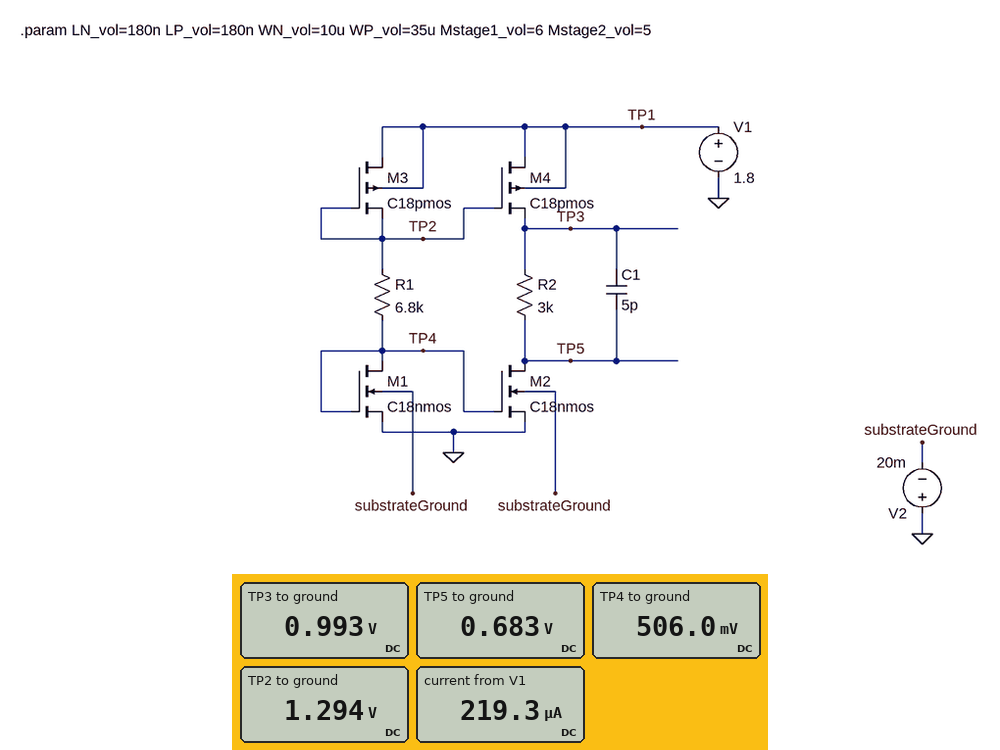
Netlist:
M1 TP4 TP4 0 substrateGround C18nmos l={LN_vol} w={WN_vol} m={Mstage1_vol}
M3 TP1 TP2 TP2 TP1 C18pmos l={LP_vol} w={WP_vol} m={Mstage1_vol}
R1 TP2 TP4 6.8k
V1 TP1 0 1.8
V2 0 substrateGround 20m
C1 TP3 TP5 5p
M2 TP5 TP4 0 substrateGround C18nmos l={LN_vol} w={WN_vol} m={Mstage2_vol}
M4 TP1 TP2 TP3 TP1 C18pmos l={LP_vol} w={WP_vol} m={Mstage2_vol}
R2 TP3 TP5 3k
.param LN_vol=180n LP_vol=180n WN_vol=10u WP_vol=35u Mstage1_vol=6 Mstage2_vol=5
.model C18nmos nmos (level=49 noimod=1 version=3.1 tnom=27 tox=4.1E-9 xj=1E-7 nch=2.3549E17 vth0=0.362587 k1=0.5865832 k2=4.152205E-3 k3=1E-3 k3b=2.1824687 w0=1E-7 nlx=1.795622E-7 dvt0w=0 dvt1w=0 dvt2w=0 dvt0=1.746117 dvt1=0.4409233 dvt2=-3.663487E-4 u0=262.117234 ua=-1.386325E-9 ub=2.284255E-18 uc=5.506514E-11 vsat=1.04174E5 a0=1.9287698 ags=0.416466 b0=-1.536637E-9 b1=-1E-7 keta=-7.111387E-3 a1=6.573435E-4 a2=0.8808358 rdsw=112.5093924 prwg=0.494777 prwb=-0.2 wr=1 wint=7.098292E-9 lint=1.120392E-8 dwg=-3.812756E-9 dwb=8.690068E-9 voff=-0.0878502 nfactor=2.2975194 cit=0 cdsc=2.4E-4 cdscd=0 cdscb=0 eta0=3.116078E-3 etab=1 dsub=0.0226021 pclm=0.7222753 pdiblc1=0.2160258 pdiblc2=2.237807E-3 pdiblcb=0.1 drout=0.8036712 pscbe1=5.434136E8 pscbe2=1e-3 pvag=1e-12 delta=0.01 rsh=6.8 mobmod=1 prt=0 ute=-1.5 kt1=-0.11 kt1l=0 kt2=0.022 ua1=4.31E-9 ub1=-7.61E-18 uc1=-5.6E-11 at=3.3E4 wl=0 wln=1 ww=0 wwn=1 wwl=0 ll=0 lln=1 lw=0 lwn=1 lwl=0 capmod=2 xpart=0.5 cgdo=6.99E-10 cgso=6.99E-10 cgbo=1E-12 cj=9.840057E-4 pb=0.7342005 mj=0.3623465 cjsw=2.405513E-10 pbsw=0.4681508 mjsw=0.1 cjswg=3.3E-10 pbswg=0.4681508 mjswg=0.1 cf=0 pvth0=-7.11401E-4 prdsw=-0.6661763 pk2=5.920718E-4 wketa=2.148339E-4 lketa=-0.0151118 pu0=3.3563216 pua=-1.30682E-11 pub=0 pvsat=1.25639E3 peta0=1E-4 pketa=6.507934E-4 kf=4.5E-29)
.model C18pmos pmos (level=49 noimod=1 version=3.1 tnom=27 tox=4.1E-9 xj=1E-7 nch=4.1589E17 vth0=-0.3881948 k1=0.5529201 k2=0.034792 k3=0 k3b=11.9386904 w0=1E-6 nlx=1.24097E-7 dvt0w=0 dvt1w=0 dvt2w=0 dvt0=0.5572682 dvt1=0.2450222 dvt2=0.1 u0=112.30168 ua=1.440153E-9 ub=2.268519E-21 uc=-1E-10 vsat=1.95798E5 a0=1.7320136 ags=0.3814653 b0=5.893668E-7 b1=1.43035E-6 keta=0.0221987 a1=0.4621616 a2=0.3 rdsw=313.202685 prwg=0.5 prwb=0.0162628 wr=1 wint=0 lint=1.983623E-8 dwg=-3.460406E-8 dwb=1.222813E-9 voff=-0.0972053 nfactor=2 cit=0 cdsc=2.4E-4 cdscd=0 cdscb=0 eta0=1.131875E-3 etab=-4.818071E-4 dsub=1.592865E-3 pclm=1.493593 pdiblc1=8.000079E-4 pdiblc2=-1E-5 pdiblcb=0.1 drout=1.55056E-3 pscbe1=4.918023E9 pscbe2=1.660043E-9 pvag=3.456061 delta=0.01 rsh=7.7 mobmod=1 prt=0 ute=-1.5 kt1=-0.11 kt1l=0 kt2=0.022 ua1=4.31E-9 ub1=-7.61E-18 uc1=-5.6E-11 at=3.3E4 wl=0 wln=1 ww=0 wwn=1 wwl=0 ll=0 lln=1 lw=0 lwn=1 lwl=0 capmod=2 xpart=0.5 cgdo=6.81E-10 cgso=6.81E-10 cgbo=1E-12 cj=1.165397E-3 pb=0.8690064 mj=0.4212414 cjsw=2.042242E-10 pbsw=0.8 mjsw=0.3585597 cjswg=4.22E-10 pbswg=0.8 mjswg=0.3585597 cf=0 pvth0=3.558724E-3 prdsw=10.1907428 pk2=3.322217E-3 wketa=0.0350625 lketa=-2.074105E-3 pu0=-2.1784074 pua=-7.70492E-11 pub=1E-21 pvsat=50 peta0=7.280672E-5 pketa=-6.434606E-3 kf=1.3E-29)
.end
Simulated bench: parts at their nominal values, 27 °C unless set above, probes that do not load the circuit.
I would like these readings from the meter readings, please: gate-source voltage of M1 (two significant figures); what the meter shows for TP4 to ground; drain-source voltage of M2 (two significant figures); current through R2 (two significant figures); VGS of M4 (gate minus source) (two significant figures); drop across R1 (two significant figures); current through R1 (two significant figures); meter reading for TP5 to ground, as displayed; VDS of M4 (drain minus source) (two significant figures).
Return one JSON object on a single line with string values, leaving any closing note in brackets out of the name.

{"gate-source voltage of M1": "510 mV", "what the meter shows for TP4 to ground": "506.0 mV", "drain-source voltage of M2": "680 mV", "current through R2": "100 µA", "VGS of M4 (gate minus source)": "300 mV", "drop across R1": "790 mV", "current through R1": "120 µA", "meter reading for TP5 to ground, as displayed": "0.683 V", "VDS of M4 (drain minus source)": "810 mV"}
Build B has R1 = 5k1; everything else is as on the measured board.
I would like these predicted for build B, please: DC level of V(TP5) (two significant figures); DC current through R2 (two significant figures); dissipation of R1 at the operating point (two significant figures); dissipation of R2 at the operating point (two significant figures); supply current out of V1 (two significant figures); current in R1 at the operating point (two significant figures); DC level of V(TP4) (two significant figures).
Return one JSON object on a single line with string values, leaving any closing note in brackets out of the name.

{"DC level of V(TP5)": "660 mV", "DC current through R2": "130 µA", "dissipation of R1 at the operating point": "110 µW", "dissipation of R2 at the operating point": "52 µW", "supply current out of V1": "280 µA", "current in R1 at the operating point": "150 µA", "DC level of V(TP4)": "520 mV"}
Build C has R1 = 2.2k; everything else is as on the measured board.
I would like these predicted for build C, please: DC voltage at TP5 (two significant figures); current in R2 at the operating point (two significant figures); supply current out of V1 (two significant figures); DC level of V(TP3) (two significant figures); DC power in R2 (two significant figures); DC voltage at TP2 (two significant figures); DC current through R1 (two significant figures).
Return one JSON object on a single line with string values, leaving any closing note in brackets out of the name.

{"DC voltage at TP5": "520 mV", "current in R2 at the operating point": "260 µA", "supply current out of V1": "570 µA", "DC level of V(TP3)": "1.3 V", "DC power in R2": "200 µW", "DC voltage at TP2": "1.2 V", "DC current through R1": "310 µA"}
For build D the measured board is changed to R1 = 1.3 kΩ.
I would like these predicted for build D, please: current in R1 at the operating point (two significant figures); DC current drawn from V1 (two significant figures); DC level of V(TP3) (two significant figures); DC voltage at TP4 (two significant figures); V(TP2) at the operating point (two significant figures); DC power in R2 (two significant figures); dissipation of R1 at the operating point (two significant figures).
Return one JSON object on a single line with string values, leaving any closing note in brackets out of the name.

{"current in R1 at the operating point": "490 µA", "DC current drawn from V1": "870 µA", "DC level of V(TP3)": "1.5 V", "DC voltage at TP4": "580 mV", "V(TP2) at the operating point": "1.2 V", "DC power in R2": "430 µW", "dissipation of R1 at the operating point": "310 µW"}
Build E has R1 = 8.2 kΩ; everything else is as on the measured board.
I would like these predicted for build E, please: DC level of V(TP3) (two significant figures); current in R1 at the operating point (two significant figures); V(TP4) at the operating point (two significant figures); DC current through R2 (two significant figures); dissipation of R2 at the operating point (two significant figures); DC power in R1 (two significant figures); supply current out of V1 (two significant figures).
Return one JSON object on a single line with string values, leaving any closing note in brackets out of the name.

{"DC level of V(TP3)": "960 mV", "current in R1 at the operating point": "98 µA", "V(TP4) at the operating point": "500 mV", "DC current through R2": "88 µA", "dissipation of R2 at the operating point": "23 µW", "DC power in R1": "79 µW", "supply current out of V1": "190 µA"}
